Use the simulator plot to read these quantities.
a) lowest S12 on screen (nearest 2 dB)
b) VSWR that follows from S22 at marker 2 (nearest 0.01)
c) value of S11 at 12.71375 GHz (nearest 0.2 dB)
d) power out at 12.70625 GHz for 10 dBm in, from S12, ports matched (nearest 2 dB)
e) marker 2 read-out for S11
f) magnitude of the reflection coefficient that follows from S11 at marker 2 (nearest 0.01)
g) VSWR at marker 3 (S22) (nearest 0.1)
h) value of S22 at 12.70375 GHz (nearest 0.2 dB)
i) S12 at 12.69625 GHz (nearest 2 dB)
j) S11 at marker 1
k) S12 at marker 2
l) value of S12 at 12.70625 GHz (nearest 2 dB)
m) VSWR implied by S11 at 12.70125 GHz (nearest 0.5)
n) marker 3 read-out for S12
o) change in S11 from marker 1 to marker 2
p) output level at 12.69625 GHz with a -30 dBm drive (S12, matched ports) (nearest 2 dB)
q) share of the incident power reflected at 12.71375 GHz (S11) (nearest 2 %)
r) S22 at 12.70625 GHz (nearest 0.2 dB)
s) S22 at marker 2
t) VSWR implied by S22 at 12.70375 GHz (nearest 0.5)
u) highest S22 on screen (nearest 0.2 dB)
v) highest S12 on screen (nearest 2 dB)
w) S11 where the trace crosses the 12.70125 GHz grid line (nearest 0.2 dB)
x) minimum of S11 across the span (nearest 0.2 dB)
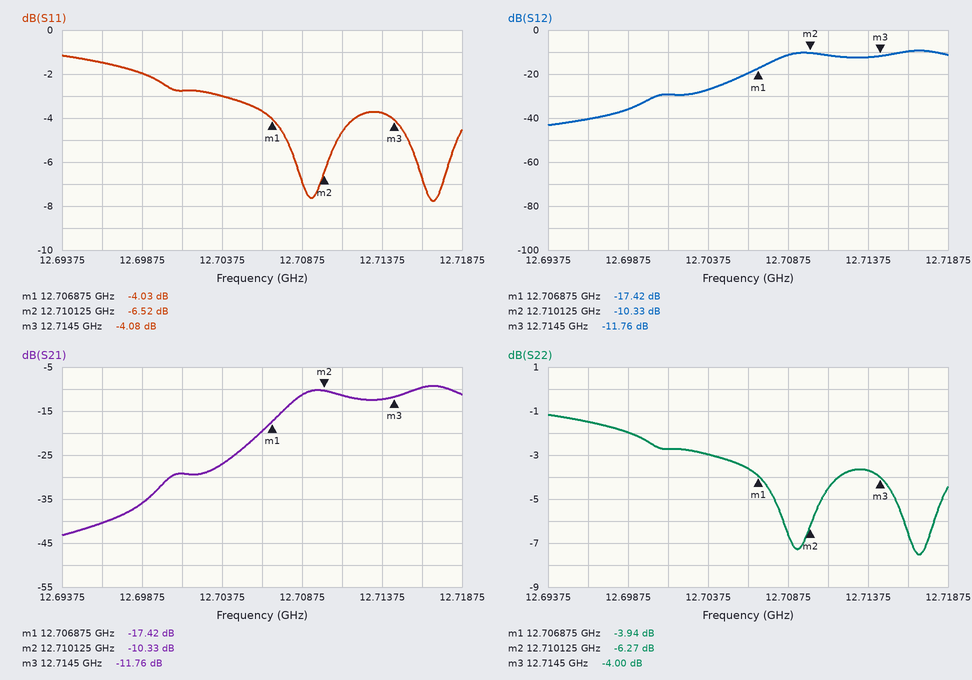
-44 dB
2.89
-3.8 dB
-10 dBm
-6.52 dB
0.47
4.4
-3.0 dB
-40 dB
-4.03 dB
-10.33 dB
-20 dB
6.5
-11.76 dB
-2.49 dB
-70 dBm
42 %
-3.6 dB
-6.27 dB
6.0
-1.2 dB
-10 dB
-2.8 dB
-7.8 dB
